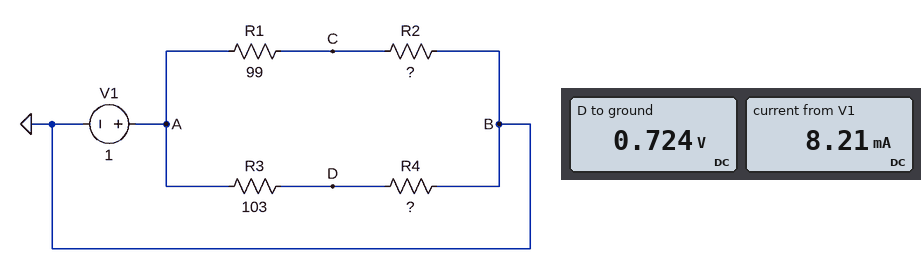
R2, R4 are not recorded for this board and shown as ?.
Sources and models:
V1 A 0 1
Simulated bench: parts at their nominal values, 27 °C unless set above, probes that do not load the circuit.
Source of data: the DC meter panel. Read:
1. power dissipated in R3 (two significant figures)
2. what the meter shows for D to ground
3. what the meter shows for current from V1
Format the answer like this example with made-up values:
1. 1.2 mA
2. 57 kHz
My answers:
1. 740 µW
2. 0.724 V
3. 8.21 mA
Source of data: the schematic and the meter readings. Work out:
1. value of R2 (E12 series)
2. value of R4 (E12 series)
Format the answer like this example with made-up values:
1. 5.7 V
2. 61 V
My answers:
1. 82 Ω
2. 270 Ω
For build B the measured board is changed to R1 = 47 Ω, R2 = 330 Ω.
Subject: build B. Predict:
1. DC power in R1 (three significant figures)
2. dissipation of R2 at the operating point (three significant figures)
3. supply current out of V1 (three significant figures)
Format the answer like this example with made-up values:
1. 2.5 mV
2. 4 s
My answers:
1. 331 µW
2. 2.32 mW
3. 5.33 mA
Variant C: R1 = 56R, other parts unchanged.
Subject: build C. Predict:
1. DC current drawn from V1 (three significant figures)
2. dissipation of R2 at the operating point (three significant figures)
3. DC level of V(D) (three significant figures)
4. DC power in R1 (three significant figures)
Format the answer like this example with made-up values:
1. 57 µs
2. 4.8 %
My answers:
1. 9.93 mA
2. 4.31 mW
3. 724 mV
4. 2.94 mW
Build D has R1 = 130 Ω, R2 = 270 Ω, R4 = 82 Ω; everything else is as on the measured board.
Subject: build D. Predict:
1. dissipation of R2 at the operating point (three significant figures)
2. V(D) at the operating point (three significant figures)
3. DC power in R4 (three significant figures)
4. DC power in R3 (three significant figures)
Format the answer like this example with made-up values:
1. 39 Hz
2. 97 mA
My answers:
1. 1.69 mW
2. 443 mV
3. 2.40 mW
4. 3.01 mW
